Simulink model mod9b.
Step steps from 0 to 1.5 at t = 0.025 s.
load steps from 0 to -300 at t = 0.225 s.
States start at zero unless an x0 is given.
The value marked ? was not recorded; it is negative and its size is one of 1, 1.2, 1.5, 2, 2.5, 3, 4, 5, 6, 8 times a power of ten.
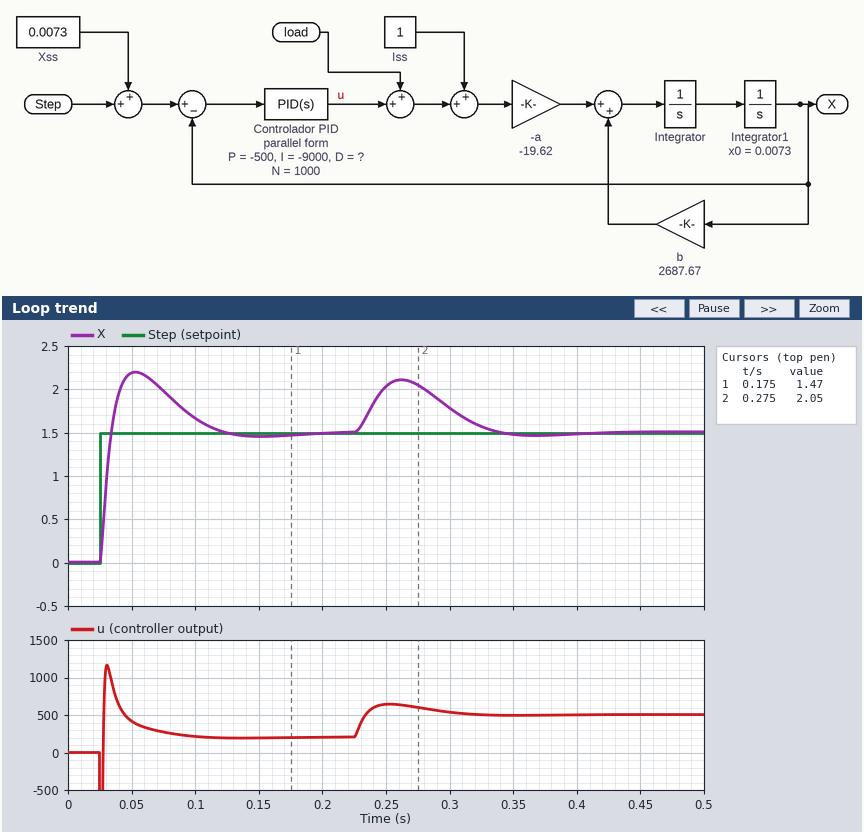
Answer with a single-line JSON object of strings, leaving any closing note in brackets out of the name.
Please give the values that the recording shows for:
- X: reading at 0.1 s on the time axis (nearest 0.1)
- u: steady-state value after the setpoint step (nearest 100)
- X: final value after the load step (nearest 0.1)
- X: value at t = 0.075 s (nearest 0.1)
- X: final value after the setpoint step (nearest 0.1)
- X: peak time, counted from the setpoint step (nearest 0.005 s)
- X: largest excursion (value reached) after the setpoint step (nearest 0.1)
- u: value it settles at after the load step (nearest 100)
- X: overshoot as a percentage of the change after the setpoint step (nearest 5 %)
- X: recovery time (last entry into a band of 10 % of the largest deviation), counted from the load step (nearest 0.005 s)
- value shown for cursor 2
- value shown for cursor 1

{"X: reading at 0.1 s on the time axis": "1.7", "u: steady-state value after the setpoint step": "200", "X: final value after the load step": "1.5", "X: value at t = 0.075 s": "2.0", "X: final value after the setpoint step": "1.5", "X: peak time, counted from the setpoint step": "0.030 s", "X: largest excursion (value reached) after the setpoint step": "2.2", "u: value it settles at after the load step": "500", "X: overshoot as a percentage of the change after the setpoint step": "45 %", "X: recovery time (last entry into a band of 10 % of the largest deviation), counted from the load step": "0.100 s", "value shown for cursor 2": "2.05", "value shown for cursor 1": "1.47"}
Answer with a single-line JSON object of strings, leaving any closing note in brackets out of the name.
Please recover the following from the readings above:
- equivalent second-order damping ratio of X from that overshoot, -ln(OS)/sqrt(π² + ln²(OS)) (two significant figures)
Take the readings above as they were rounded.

{"equivalent second-order damping ratio of X from that overshoot, -ln(OS)/sqrt(π² + ln²(OS))": "0.25"}
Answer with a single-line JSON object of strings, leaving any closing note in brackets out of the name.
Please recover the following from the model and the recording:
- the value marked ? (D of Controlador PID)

{"the value marked ?": "-8"}
